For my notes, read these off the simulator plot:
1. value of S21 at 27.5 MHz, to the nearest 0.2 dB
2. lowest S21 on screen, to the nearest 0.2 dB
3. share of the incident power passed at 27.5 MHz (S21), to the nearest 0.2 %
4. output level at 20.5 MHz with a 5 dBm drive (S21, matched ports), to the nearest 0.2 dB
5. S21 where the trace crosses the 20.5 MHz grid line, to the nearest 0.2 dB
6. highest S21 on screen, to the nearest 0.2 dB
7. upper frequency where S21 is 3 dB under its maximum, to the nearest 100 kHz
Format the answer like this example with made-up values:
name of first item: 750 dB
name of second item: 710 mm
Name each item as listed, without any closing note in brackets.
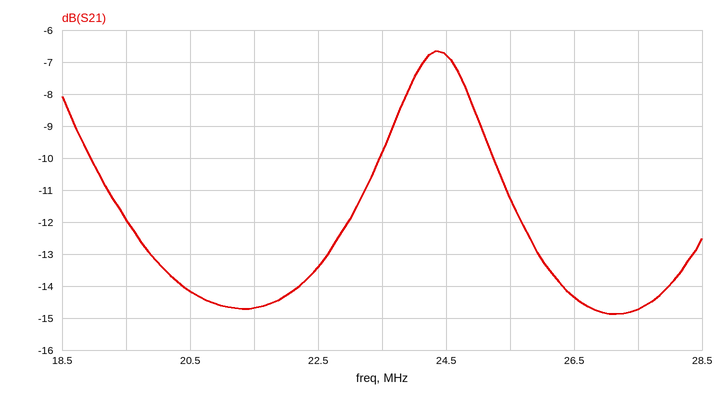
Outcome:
value of S21 at 27.5 MHz, to the nearest 0.2 dB: -14.8 dB
lowest S21 on screen, to the nearest 0.2 dB: -14.8 dB
share of the incident power passed at 27.5 MHz (S21), to the nearest 0.2 %: 3.4 %
output level at 20.5 MHz with a 5 dBm drive (S21, matched ports), to the nearest 0.2 dB: -9.2 dBm
S21 where the trace crosses the 20.5 MHz grid line, to the nearest 0.2 dB: -14.2 dB
highest S21 on screen, to the nearest 0.2 dB: -6.6 dB
upper frequency where S21 is 3 dB under its maximum, to the nearest 100 kHz: 25.2 MHz
